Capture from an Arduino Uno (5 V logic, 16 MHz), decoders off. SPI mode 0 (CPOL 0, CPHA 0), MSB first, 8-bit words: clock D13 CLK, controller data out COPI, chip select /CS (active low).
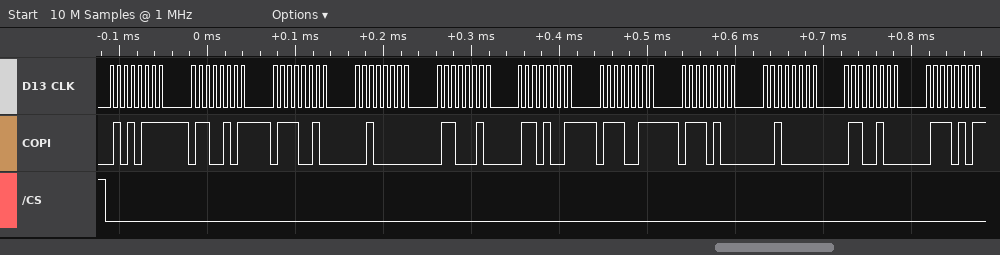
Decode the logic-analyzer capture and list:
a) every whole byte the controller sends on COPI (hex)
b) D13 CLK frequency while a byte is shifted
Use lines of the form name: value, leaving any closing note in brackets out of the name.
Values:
every whole byte the controller sends on COPI: 0x57 0x65 0x72 0x20 0x62 0x69 0x73 0x74 0x20 0x64 0x75
D13 CLK frequency while a byte is shifted: 125 kHz
